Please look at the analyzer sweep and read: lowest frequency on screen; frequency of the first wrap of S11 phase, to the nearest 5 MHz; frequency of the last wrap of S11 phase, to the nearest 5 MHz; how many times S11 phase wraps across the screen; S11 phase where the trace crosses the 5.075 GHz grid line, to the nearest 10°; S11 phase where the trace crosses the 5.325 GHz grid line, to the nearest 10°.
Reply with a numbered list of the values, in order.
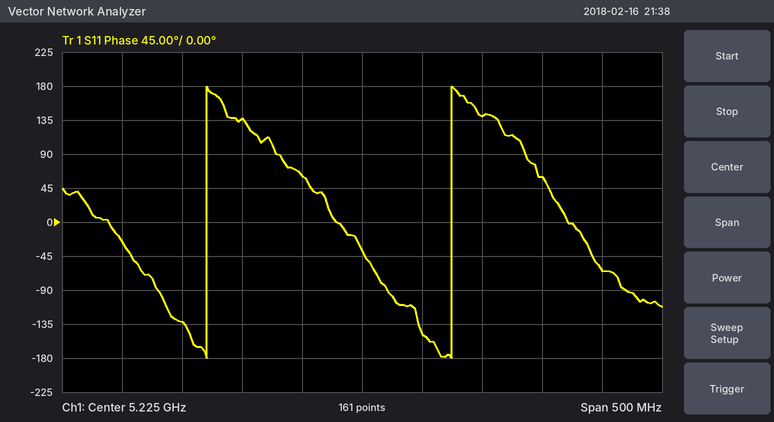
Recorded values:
1. 4.975 GHz
2. 5.095 GHz
3. 5.300 GHz
4. 2
5. -130°
6. 140°
